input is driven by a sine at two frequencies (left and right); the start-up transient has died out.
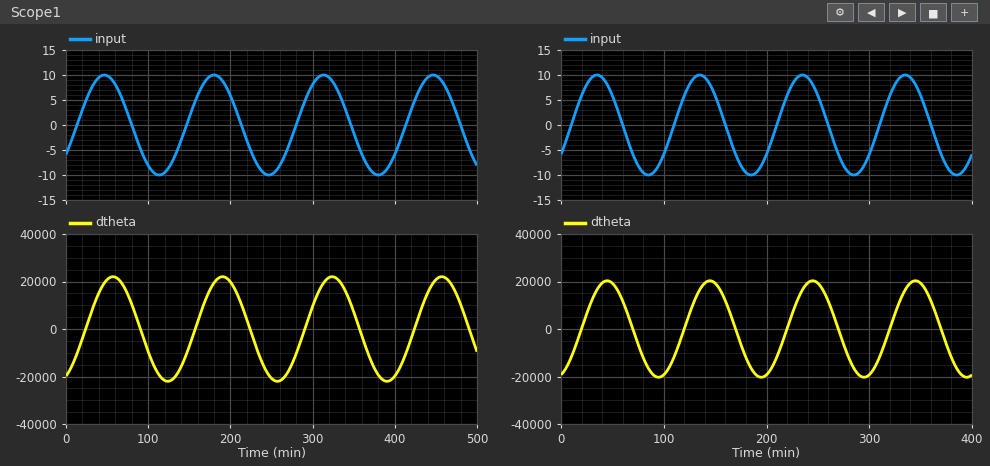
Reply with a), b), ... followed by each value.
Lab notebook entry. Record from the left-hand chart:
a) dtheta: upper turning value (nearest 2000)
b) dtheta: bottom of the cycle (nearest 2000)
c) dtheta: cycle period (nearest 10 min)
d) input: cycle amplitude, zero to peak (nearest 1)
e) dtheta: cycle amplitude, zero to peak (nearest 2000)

a) 22000
b) -22000
c) 130 min
d) 10
e) 22000
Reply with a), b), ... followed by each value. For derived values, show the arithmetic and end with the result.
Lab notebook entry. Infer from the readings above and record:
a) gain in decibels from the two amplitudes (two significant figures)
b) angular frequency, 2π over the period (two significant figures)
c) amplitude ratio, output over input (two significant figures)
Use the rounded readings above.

a) 20 log10(22000 / 10) = 67 dB
b) 2π / 130 = 0.048 rad/min
c) 22000 / 10 = 2200
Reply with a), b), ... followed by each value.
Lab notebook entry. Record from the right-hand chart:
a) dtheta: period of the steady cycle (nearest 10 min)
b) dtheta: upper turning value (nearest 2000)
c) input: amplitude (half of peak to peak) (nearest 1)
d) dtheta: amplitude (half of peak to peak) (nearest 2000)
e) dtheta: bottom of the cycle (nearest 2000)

a) 100 min
b) 20000
c) 10
d) 20000
e) -20000
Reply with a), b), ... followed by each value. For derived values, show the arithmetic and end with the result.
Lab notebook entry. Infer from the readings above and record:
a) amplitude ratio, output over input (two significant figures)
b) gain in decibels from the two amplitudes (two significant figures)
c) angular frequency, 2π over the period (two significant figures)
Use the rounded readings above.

a) 20000 / 10 = 2000
b) 20 log10(20000 / 10) = 66 dB
c) 2π / 100 = 0.063 rad/min
